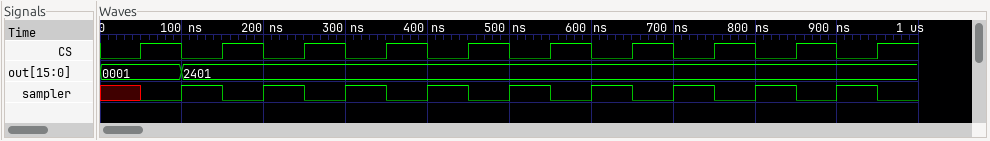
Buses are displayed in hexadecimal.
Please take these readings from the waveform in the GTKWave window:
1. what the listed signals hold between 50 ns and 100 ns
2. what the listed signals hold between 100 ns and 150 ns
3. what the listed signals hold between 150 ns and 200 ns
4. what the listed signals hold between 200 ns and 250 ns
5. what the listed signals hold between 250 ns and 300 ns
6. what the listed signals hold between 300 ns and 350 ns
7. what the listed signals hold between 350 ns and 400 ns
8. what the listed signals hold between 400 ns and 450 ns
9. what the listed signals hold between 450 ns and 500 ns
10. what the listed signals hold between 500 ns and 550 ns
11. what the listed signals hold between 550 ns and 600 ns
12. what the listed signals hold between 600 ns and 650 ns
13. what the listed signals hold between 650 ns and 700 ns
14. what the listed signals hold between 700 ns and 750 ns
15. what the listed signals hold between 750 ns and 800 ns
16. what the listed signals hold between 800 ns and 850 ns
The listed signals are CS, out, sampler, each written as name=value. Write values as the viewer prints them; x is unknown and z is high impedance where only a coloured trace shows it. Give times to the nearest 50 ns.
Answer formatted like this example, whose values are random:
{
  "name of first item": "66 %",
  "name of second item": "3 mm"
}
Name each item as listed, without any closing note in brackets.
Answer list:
{
  "what the listed signals hold between 50 ns and 100 ns": "CS=1, out=0001, sampler=0",
  "what the listed signals hold between 100 ns and 150 ns": "CS=0, out=2401, sampler=1",
  "what the listed signals hold between 150 ns and 200 ns": "CS=1, out=2401, sampler=0",
  "what the listed signals hold between 200 ns and 250 ns": "CS=0, out=2401, sampler=1",
  "what the listed signals hold between 250 ns and 300 ns": "CS=1, out=2401, sampler=0",
  "what the listed signals hold between 300 ns and 350 ns": "CS=0, out=2401, sampler=1",
  "what the listed signals hold between 350 ns and 400 ns": "CS=1, out=2401, sampler=0",
  "what the listed signals hold between 400 ns and 450 ns": "CS=0, out=2401, sampler=1",
  "what the listed signals hold between 450 ns and 500 ns": "CS=1, out=2401, sampler=0",
  "what the listed signals hold between 500 ns and 550 ns": "CS=0, out=2401, sampler=1",
  "what the listed signals hold between 550 ns and 600 ns": "CS=1, out=2401, sampler=0",
  "what the listed signals hold between 600 ns and 650 ns": "CS=0, out=2401, sampler=1",
  "what the listed signals hold between 650 ns and 700 ns": "CS=1, out=2401, sampler=0",
  "what the listed signals hold between 700 ns and 750 ns": "CS=0, out=2401, sampler=1",
  "what the listed signals hold between 750 ns and 800 ns": "CS=1, out=2401, sampler=0",
  "what the listed signals hold between 800 ns and 850 ns": "CS=0, out=2401, sampler=1"
}
